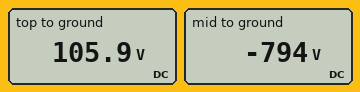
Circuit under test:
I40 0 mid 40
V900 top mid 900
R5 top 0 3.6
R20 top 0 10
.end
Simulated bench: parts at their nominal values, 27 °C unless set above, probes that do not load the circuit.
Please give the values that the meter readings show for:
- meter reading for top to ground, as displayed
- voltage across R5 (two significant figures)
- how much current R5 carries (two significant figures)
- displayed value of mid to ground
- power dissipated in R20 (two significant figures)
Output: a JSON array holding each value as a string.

["105.9 V", "110 V", "29 A", "-794 V", "1.1 kW"]
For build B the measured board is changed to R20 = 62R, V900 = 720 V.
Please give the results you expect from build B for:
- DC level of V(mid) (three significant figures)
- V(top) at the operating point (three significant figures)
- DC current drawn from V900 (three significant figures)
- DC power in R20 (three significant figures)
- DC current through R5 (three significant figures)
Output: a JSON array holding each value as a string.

["-584 V", "136 V", "40.0 A", "299 W", "37.8 A"]
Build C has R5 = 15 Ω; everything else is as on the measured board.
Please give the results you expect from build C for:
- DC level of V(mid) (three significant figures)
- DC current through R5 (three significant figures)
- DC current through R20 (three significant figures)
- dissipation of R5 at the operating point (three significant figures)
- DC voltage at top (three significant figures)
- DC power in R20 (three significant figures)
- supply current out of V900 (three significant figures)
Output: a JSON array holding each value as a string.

["-660 V", "16.0 A", "24.0 A", "3.84 kW", "240 V", "5.76 kW", "40.0 A"]
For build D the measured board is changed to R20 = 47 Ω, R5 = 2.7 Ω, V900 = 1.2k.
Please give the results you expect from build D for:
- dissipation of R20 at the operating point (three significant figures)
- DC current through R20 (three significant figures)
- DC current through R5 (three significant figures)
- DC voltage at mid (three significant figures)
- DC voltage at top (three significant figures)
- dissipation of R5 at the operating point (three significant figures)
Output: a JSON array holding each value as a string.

["222 W", "2.17 A", "37.8 A", "-1.10 kV", "102 V", "3.86 kW"]
